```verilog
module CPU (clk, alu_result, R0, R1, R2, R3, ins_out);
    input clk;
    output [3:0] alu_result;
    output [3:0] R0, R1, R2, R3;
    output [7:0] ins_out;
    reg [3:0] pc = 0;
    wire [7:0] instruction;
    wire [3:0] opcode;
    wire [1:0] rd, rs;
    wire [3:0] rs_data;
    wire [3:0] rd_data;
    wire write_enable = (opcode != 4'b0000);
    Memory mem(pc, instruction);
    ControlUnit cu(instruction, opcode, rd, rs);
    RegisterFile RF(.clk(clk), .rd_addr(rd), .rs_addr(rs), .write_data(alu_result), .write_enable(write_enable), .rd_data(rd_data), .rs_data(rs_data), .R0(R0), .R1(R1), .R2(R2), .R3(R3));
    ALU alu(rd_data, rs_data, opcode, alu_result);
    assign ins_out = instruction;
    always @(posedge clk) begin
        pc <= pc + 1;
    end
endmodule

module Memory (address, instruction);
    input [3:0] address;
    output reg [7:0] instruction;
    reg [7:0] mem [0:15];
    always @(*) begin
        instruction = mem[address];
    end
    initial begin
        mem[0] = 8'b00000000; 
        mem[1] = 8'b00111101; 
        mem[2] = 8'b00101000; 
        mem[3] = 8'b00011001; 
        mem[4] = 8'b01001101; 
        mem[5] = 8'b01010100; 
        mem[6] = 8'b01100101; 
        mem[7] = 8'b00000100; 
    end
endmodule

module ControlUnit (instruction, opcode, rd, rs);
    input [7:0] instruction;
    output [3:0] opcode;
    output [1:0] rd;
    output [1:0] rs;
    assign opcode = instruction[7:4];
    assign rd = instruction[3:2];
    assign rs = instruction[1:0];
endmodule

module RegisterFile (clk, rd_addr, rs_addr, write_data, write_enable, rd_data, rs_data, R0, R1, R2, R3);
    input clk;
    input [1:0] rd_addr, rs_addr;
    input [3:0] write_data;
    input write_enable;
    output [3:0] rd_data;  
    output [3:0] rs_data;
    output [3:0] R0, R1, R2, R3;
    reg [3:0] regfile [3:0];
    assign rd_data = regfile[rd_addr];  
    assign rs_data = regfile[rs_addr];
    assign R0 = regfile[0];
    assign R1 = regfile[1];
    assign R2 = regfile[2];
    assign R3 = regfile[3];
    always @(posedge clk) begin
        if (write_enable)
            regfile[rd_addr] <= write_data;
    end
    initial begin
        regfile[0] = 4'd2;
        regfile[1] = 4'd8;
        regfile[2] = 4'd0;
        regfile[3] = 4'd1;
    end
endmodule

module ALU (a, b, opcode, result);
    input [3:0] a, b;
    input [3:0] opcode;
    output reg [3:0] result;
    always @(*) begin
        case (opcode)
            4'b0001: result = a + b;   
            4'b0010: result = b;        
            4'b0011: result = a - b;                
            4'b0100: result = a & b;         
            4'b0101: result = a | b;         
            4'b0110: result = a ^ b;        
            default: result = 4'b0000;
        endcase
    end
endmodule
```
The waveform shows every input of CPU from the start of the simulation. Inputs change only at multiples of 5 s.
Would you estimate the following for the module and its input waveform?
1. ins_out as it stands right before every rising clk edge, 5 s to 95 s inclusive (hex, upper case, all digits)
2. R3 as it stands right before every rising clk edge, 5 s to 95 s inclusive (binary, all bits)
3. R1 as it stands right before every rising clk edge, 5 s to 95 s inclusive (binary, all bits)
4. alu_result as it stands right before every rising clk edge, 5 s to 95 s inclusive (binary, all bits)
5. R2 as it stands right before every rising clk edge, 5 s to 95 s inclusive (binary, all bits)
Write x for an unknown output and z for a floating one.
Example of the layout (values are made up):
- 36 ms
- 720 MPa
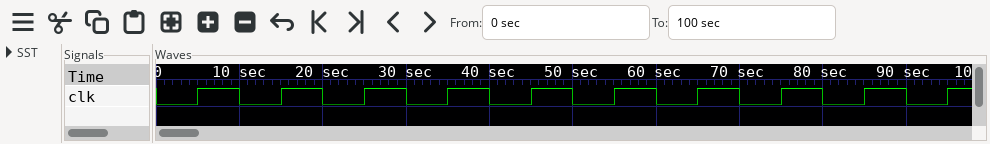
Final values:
- 00, 3D, 28, 19, 4D, 54, 65, 04, x, x
- 0001, 0001, 1001, 1001, 1001, 1000, 1000, 1000, 1000, 1000
- 1000, 1000, 1000, 1000, 1000, 1000, 1010, 0000, 0000, 0000
- 0000, 1001, 0010, 1010, 1000, 1010, 0000, 0000, 0000, 0000
- 0000, 0000, 0000, 0010, 1010, 1010, 1010, 1010, 1010, 1010
